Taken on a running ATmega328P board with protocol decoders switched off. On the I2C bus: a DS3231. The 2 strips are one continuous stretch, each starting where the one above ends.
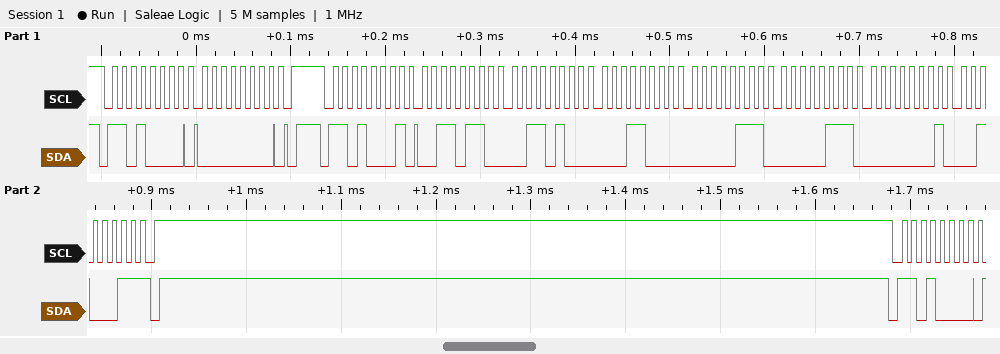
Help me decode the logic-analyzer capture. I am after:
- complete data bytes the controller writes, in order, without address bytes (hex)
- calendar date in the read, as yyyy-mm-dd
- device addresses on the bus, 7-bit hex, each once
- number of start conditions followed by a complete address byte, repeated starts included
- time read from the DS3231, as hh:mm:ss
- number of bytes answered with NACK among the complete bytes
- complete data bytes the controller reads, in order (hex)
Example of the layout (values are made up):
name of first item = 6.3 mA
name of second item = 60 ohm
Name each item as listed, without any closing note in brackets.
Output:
complete data bytes the controller writes, in order, without address bytes = 00
calendar date in the read, as yyyy-mm-dd = 2023-01-07
device addresses on the bus, 7-bit hex, each once = 0x68
number of start conditions followed by a complete address byte, repeated starts included = 3
time read from the DS3231, as hh:mm:ss = 18:34:36
number of bytes answered with NACK among the complete bytes = 1
complete data bytes the controller reads, in order = 36 34 18 07 07 01 23
